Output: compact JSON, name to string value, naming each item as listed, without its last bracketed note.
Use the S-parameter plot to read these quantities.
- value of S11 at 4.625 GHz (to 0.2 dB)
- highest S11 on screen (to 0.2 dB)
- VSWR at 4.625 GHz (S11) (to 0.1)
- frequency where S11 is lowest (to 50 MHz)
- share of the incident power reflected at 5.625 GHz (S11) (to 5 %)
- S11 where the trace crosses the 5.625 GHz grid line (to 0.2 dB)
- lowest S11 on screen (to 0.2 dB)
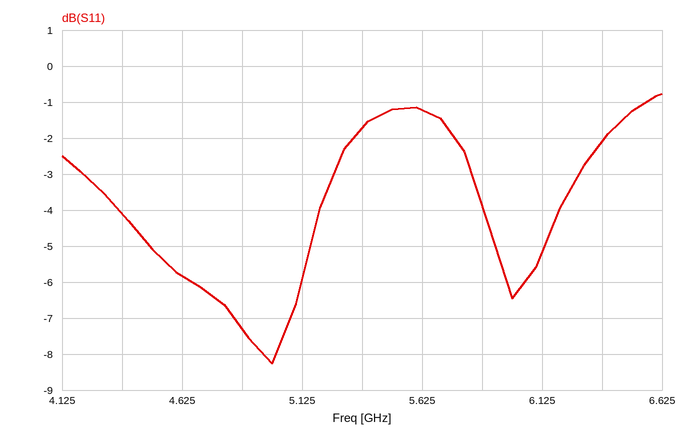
{"value of S11 at 4.625 GHz": "-5.8 dB", "highest S11 on screen": "-0.8 dB", "VSWR at 4.625 GHz (S11)": "3.1", "frequency where S11 is lowest": "5.00 GHz", "share of the incident power reflected at 5.625 GHz (S11)": "75 %", "S11 where the trace crosses the 5.625 GHz grid line": "-1.2 dB", "lowest S11 on screen": "-8.2 dB"}
